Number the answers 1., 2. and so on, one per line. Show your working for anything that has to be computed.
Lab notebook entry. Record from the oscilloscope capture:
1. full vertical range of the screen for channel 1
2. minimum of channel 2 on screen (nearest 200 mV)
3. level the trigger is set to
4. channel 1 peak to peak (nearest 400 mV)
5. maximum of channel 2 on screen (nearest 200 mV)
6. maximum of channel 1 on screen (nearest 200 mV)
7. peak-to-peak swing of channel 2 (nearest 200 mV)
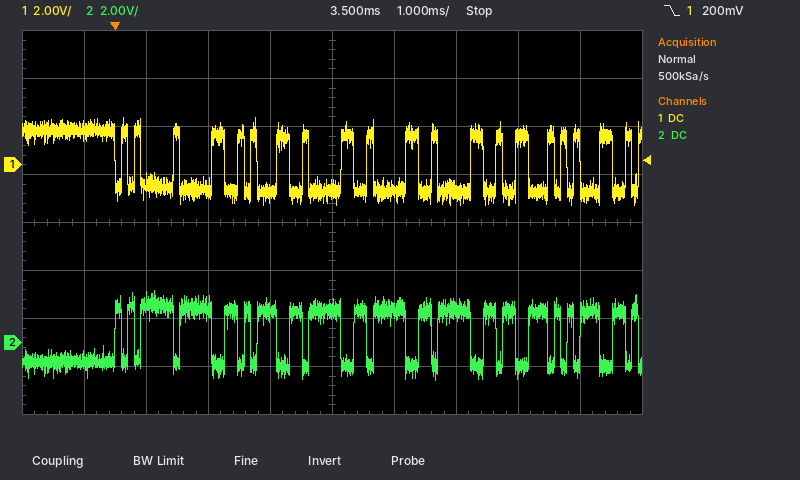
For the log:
1. 16 V
2. -1.6 V
3. 200 mV
4. 3.6 V
5. 2.2 V
6. 2.0 V
7. 2.2 V − (-1.6 V) = 3.8 V
